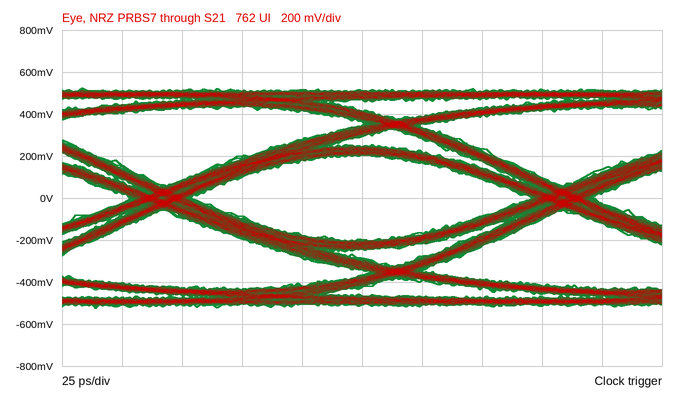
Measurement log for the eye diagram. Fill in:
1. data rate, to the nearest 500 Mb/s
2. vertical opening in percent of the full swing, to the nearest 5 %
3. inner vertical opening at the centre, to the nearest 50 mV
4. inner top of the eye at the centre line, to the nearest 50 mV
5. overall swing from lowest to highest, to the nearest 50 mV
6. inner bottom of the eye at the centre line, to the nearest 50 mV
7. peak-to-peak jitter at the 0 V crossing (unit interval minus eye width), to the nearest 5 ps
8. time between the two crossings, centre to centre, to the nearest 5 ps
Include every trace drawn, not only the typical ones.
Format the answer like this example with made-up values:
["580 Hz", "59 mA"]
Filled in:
["6.0 Gb/s", "40 %", "400 mV", "200 mV", "1.05 V", "-200 mV", "25 ps", "165 ps"]
